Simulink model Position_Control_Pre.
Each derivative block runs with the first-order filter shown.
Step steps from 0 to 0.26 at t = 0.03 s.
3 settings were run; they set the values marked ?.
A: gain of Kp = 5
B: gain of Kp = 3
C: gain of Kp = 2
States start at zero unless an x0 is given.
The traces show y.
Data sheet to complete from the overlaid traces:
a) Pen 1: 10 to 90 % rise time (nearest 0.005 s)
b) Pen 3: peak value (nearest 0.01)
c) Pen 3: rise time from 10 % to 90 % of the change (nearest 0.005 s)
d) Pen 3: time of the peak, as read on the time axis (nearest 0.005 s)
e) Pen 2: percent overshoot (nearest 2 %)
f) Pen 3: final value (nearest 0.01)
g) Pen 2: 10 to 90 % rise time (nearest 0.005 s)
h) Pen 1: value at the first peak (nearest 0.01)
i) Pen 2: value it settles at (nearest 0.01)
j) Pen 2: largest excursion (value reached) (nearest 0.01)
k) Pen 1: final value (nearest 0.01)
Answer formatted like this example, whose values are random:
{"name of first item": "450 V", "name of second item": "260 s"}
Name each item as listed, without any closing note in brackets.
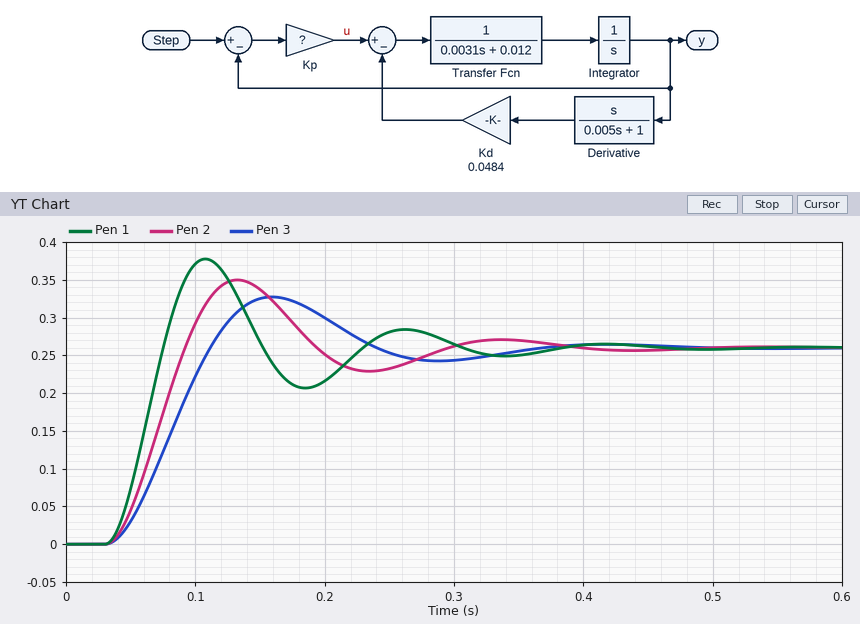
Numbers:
{"Pen 1: 10 to 90 % rise time": "0.030 s", "Pen 3: peak value": "0.33", "Pen 3: rise time from 10 % to 90 % of the change": "0.055 s", "Pen 3: time of the peak, as read on the time axis": "0.160 s", "Pen 2: percent overshoot": "34 %", "Pen 3: final value": "0.26", "Pen 2: 10 to 90 % rise time": "0.040 s", "Pen 1: value at the first peak": "0.38", "Pen 2: value it settles at": "0.26", "Pen 2: largest excursion (value reached)": "0.35", "Pen 1: final value": "0.26"}
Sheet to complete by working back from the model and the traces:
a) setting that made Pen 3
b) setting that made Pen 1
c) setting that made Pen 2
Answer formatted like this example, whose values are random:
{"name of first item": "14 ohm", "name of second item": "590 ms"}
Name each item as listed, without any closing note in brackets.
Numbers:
{"setting that made Pen 3": "C", "setting that made Pen 1": "A", "setting that made Pen 2": "B"}
